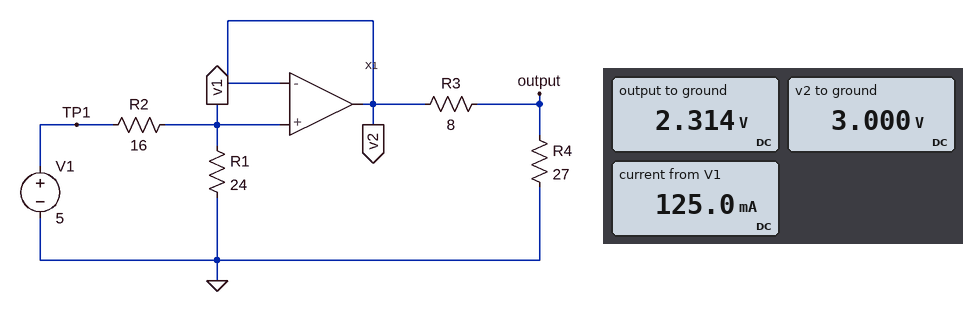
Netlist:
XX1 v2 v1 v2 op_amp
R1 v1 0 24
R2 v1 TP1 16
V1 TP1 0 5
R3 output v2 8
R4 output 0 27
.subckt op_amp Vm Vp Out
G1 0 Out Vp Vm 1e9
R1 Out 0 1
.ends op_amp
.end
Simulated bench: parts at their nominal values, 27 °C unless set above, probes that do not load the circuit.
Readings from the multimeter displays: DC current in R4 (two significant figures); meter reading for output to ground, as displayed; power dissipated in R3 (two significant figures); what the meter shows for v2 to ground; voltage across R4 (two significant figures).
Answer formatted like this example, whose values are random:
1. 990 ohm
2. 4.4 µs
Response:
1. 86 mA
2. 2.314 V
3. 59 mW
4. 3.000 V
5. 2.3 V
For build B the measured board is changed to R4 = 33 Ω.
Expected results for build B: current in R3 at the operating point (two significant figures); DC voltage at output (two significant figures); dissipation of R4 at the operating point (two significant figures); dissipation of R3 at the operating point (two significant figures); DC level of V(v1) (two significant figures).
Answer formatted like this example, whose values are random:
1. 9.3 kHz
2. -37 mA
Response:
1. 73 mA
2. 2.4 V
3. 180 mW
4. 43 mW
5. 3.0 V
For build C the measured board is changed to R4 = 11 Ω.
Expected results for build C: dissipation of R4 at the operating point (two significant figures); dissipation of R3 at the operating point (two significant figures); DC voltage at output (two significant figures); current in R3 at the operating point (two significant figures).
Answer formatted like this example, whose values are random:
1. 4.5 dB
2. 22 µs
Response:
1. 270 mW
2. 200 mW
3. 1.7 V
4. 160 mA
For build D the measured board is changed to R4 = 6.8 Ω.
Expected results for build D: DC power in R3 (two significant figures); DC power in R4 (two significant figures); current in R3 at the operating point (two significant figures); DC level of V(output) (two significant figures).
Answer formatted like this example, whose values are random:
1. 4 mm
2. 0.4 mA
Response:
1. 330 mW
2. 280 mW
3. 200 mA
4. 1.4 V
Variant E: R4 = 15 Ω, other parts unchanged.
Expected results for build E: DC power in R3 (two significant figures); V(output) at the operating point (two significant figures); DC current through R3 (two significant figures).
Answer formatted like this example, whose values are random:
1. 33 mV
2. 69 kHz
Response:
1. 140 mW
2. 2.0 V
3. 130 mA
